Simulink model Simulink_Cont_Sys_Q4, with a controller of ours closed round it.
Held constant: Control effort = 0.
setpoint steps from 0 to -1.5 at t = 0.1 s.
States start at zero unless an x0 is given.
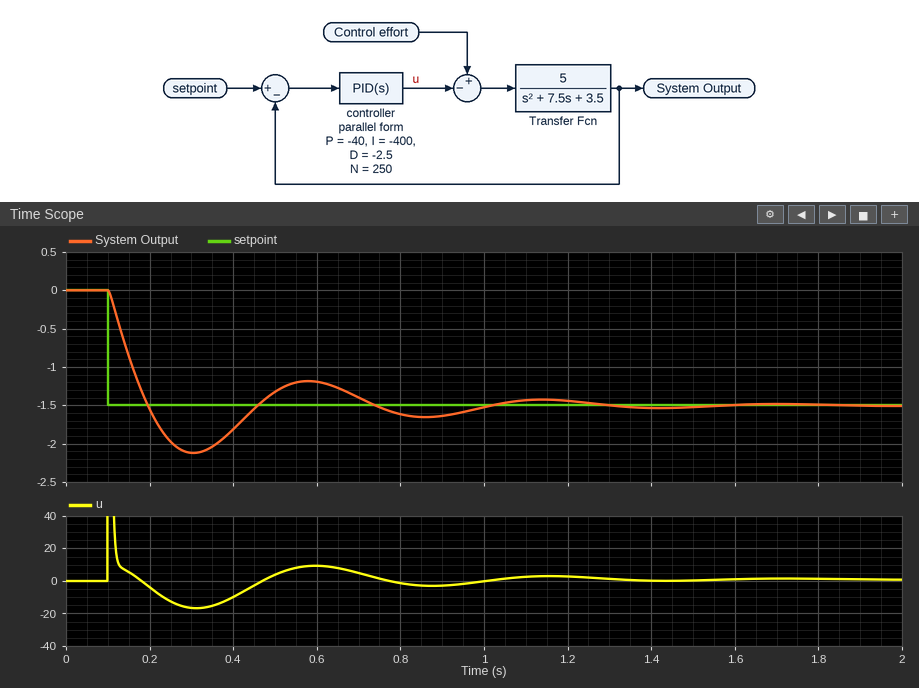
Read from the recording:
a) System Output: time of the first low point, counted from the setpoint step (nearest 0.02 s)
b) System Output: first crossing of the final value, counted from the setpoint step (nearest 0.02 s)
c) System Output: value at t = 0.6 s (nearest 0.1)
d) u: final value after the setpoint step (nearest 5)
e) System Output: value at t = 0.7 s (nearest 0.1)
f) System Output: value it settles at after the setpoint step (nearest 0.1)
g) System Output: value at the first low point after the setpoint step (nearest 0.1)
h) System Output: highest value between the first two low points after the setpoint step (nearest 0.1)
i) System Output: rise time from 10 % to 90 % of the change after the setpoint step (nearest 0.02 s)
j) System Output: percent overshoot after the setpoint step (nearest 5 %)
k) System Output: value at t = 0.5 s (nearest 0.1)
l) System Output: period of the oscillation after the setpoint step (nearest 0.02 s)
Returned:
0.20 s
0.10 s
-1.2
0
-1.4
-1.5
-2.1
-1.2
0.08 s
40 %
-1.3
0.56 s
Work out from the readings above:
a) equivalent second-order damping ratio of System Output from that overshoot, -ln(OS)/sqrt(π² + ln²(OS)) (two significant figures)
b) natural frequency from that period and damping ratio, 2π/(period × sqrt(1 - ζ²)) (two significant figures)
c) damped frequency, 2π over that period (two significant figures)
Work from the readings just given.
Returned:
0.28
12 rad/s
11 rad/s
